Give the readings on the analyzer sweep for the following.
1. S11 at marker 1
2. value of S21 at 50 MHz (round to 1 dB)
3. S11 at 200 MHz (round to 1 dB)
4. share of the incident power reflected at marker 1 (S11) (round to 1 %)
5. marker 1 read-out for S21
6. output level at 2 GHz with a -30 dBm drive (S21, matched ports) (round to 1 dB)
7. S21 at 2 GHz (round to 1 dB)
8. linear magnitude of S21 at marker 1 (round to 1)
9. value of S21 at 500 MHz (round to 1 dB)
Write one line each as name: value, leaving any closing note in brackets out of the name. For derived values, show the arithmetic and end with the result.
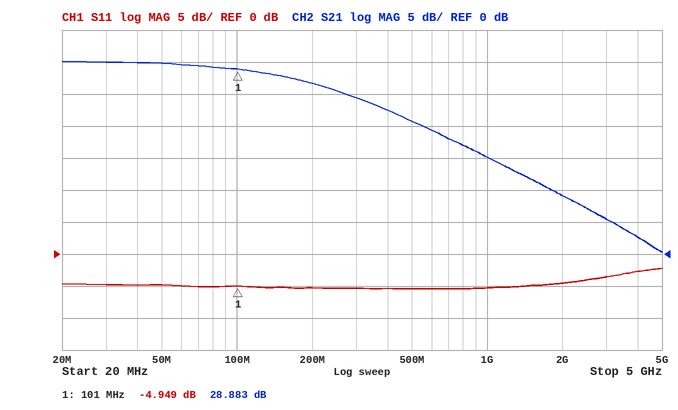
S11 at marker 1: -4.949 dB
value of S21 at 50 MHz: 30 dB
S11 at 200 MHz: -5 dB
share of the incident power reflected at marker 1 (S11): 10^(-4.949/10) ≈ 32 %
marker 1 read-out for S21: 28.883 dB
output level at 2 GHz with a -30 dBm drive (S21, matched ports): -30 dBm + (9 dB) = -21 dBm
S21 at 2 GHz: 9 dB
linear magnitude of S21 at marker 1: 10^(28.883/20) ≈ 28
value of S21 at 500 MHz: 21 dB
